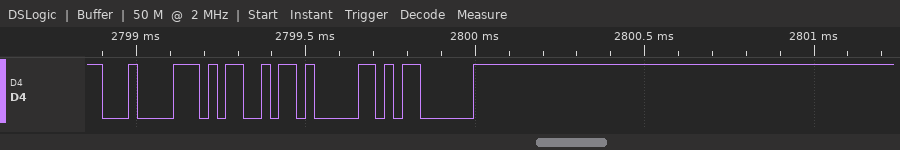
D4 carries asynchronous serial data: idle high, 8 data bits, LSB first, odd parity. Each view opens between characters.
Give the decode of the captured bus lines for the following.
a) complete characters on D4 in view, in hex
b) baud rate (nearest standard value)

84, 4D, C1, 03
38400 baud
